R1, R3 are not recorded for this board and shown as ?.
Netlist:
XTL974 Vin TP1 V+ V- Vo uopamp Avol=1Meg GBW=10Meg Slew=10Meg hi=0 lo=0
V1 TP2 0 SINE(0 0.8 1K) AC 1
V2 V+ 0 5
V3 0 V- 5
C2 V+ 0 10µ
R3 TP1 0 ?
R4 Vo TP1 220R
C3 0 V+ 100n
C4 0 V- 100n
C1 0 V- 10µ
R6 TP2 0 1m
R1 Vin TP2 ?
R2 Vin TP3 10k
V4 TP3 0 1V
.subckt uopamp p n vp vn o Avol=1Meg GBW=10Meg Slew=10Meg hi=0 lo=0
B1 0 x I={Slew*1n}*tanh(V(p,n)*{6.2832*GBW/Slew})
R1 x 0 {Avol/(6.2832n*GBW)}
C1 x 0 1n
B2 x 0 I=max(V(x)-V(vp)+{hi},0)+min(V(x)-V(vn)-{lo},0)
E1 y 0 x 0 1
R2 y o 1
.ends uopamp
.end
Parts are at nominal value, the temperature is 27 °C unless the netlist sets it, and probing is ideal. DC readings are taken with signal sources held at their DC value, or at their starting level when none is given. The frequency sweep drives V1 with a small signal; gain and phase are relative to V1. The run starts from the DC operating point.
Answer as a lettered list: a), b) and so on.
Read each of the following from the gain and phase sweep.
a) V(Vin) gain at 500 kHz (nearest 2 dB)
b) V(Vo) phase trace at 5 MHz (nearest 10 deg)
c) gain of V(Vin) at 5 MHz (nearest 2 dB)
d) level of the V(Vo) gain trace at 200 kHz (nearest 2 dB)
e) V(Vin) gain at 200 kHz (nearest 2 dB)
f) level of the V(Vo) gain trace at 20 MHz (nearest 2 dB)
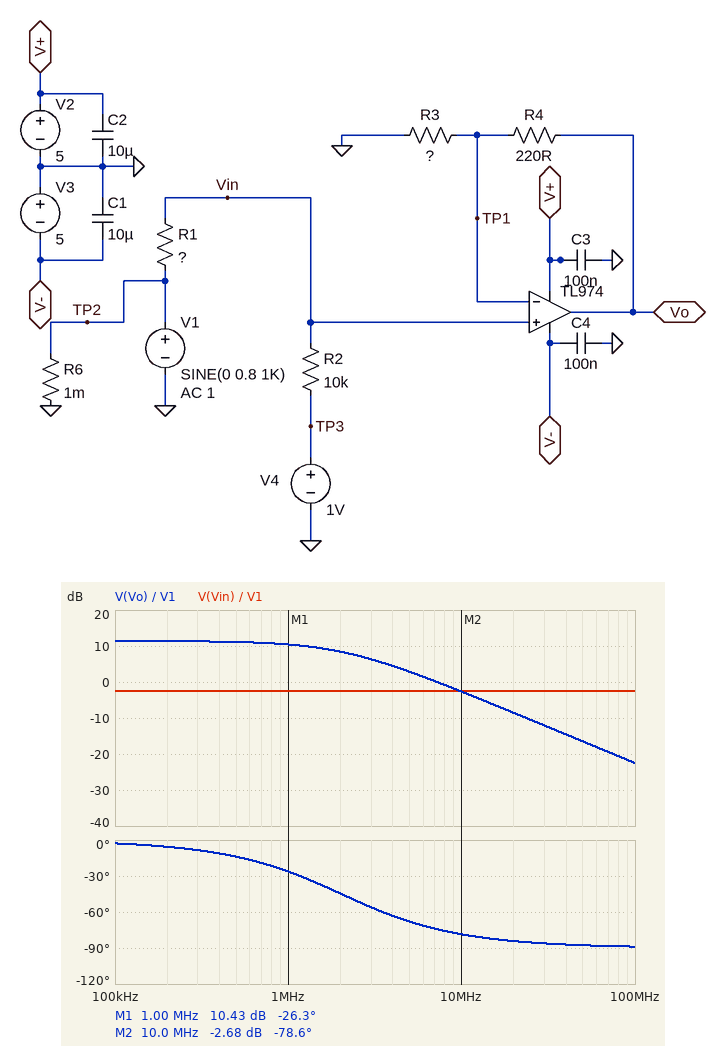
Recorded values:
a) -2 dB
b) -70 deg
c) -2 dB
d) 12 dB
e) -2 dB
f) -8 dB
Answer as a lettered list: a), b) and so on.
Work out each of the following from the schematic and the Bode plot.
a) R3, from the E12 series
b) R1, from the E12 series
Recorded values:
a) 56 Ω
b) 3.3 kΩ
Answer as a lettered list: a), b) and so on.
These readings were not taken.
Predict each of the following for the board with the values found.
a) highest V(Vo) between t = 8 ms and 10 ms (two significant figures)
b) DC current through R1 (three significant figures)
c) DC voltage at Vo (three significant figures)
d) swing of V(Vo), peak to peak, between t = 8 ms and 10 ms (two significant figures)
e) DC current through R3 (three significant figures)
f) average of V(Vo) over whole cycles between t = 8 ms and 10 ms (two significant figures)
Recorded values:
a) 4.2 V
b) 75.2 µA
c) 1.22 V
d) 5.9 V
e) 4.43 mA
f) 1.2 V
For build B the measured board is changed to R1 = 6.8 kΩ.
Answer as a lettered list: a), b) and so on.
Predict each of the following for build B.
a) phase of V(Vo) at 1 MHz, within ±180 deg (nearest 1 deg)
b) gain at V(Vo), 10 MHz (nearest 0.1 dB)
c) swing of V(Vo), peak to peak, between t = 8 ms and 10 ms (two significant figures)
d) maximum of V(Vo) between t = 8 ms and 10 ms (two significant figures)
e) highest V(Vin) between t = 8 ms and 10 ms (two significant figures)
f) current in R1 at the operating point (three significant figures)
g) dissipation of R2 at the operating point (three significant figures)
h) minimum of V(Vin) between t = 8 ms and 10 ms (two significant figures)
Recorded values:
a) -26 deg
b) -4.7 dB
c) 4.7 V
d) 4.3 V
e) 880 mV
f) 59.5 µA
g) 35.4 µW
h) -71 mV
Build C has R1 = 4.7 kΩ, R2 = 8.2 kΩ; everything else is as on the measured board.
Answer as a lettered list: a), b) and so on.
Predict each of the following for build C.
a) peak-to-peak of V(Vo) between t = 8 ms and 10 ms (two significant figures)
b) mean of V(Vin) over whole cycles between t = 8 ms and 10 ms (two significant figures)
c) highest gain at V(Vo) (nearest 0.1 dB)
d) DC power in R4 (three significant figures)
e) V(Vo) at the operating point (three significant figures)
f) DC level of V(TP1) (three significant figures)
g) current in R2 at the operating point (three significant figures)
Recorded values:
a) 5.0 V
b) 360 mV
c) 9.9 dB
d) 9.31 mW
e) 1.80 V
f) 364 mV
g) 77.5 µA
